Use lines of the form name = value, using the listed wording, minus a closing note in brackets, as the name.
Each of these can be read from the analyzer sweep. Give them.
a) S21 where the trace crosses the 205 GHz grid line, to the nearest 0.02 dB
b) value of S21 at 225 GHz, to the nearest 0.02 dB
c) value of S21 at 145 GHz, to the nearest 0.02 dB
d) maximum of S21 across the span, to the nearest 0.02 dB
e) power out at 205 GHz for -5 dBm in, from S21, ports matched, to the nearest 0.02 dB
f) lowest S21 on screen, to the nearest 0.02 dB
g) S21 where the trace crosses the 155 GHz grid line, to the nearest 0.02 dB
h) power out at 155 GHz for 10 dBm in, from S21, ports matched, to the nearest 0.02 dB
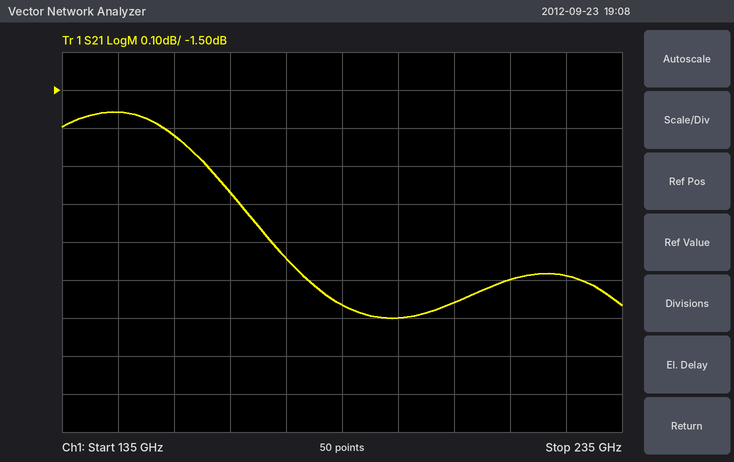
S21 where the trace crosses the 205 GHz grid line, to the nearest 0.02 dB = -2.06 dB
value of S21 at 225 GHz, to the nearest 0.02 dB = -1.98 dB
value of S21 at 145 GHz, to the nearest 0.02 dB = -1.56 dB
maximum of S21 across the span, to the nearest 0.02 dB = -1.56 dB
power out at 205 GHz for -5 dBm in, from S21, ports matched, to the nearest 0.02 dB = -7.06 dBm
lowest S21 on screen, to the nearest 0.02 dB = -2.10 dB
S21 where the trace crosses the 155 GHz grid line, to the nearest 0.02 dB = -1.62 dB
power out at 155 GHz for 10 dBm in, from S21, ports matched, to the nearest 0.02 dB = 8.38 dBm
